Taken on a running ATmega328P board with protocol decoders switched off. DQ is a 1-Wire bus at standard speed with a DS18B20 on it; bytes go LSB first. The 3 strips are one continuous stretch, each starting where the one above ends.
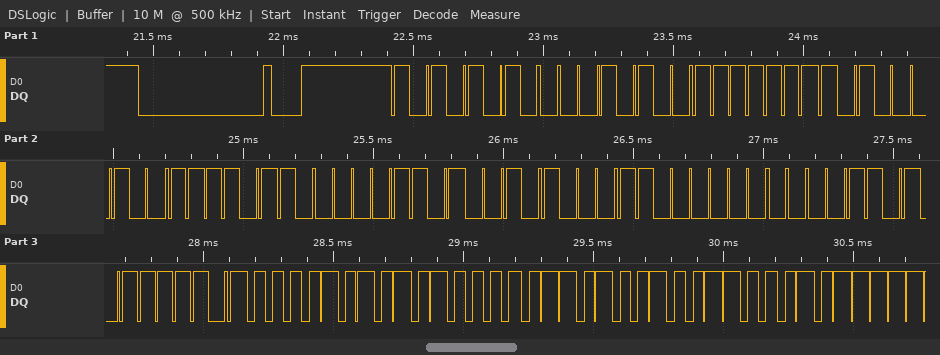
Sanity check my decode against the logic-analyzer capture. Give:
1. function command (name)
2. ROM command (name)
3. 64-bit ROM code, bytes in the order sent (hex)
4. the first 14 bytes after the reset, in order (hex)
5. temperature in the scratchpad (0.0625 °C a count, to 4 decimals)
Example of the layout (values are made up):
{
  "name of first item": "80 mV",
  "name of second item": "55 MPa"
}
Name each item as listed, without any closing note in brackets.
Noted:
{
  "function command": "Read Scratchpad",
  "ROM command": "Match ROM",
  "64-bit ROM code, bytes in the order sent": "28 FF 22 6F B0 14 03 B0",
  "the first 14 bytes after the reset, in order": "55 28 FF 22 6F B0 14 03 B0 BE 50 05 4B 46",
  "temperature in the scratchpad": "85.0000 °C"
}
